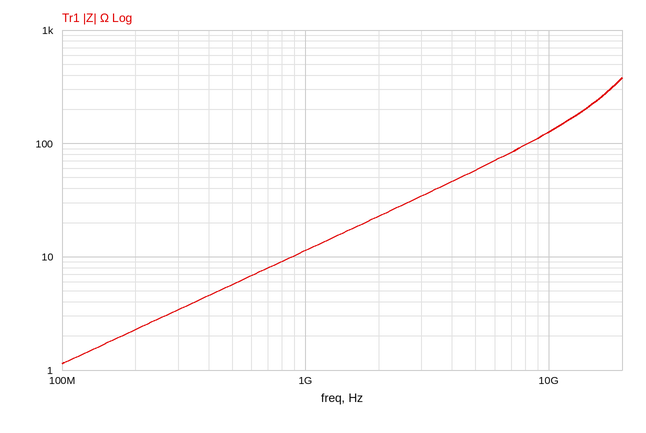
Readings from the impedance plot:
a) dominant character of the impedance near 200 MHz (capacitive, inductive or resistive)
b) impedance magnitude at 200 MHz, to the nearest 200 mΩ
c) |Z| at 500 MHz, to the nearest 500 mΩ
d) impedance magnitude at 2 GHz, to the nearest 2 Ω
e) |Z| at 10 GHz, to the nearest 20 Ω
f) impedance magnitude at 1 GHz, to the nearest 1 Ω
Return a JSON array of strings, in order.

["inductive", "2.2 Ω", "5.5 Ω", "22 Ω", "120 Ω", "11 Ω"]
